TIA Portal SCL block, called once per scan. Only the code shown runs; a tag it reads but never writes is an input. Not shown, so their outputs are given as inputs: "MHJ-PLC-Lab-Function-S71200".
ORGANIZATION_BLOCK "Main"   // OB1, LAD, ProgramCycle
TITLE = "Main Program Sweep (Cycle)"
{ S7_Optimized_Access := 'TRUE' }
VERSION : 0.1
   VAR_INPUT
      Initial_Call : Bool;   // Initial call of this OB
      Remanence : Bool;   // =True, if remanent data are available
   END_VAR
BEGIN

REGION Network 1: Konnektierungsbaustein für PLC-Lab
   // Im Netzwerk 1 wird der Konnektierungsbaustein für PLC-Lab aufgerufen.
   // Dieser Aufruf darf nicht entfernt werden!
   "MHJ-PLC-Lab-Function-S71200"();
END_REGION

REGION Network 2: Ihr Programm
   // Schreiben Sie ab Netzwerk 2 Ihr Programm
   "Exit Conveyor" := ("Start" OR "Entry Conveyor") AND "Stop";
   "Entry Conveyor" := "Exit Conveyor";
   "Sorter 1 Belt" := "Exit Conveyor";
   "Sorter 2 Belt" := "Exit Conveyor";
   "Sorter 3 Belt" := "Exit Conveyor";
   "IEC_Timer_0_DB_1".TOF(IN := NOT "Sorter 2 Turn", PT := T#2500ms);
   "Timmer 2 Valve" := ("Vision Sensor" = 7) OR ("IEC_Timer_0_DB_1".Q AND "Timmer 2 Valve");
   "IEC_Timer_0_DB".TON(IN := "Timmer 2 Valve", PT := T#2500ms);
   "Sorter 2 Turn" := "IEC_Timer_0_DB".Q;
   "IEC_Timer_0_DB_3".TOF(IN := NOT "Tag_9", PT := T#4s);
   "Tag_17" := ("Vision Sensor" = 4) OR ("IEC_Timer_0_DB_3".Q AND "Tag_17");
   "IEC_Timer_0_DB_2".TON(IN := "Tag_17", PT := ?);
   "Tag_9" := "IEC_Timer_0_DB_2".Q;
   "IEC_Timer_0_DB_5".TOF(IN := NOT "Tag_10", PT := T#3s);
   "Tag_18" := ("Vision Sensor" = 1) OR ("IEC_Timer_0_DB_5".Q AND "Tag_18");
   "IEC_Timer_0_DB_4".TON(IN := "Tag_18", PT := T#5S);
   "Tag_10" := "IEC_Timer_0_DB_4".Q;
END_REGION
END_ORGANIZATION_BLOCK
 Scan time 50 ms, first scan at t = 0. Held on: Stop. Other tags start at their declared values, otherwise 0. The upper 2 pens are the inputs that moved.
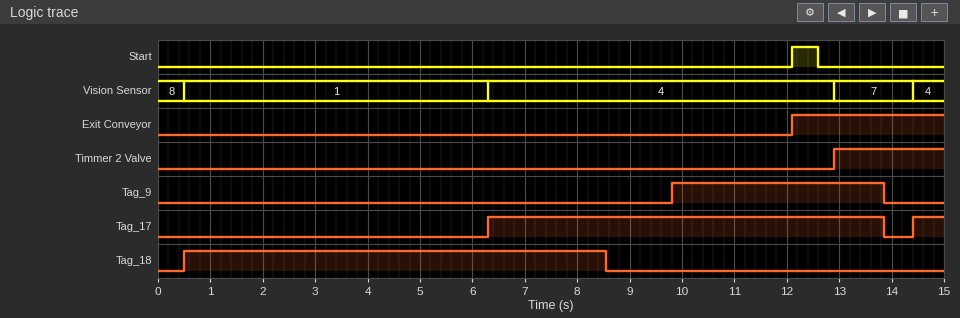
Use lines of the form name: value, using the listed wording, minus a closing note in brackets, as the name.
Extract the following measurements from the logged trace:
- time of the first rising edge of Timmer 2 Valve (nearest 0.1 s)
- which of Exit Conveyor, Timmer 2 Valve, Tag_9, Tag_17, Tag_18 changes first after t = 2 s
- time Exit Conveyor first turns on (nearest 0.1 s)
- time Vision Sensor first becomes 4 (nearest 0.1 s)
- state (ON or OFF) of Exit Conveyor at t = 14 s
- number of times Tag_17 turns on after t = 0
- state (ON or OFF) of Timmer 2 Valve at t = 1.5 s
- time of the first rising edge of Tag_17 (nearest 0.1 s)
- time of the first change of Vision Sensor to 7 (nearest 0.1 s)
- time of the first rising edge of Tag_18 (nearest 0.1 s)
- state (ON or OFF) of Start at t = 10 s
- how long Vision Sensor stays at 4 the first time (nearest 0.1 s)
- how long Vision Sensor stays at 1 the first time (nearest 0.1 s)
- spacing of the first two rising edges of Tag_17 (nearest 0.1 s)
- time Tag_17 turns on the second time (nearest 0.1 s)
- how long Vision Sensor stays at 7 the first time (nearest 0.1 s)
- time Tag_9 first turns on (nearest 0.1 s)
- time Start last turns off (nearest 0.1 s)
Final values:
time of the first rising edge of Timmer 2 Valve: 12.9 s
which of Exit Conveyor, Timmer 2 Valve, Tag_9, Tag_17, Tag_18 changes first after t = 2 s: Tag_17
time Exit Conveyor first turns on: 12.1 s
time Vision Sensor first becomes 4: 6.3 s
state (ON or OFF) of Exit Conveyor at t = 14 s: ON
number of times Tag_17 turns on after t = 0: 2
state (ON or OFF) of Timmer 2 Valve at t = 1.5 s: OFF
time of the first rising edge of Tag_17: 6.3 s
time of the first change of Vision Sensor to 7: 12.9 s
time of the first rising edge of Tag_18: 0.5 s
state (ON or OFF) of Start at t = 10 s: OFF
how long Vision Sensor stays at 4 the first time: 6.6 s
how long Vision Sensor stays at 1 the first time: 5.8 s
spacing of the first two rising edges of Tag_17: 8.1 s
time Tag_17 turns on the second time: 14.4 s
how long Vision Sensor stays at 7 the first time: 1.5 s
time Tag_9 first turns on: 9.8 s
time Start last turns off: 12.6 s
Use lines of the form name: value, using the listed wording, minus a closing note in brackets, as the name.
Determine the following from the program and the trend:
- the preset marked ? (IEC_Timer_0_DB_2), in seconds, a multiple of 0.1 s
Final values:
the preset marked ? (IEC_Timer_0_DB_2), in seconds, a multiple of 0.1 s: 3.5 s
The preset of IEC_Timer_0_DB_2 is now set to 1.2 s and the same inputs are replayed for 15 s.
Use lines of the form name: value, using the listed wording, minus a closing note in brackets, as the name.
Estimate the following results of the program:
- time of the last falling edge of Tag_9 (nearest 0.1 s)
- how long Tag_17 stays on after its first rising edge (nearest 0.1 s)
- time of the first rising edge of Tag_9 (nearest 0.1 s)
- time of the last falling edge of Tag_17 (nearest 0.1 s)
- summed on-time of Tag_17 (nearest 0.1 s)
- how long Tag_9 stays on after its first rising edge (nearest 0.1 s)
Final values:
time of the last falling edge of Tag_9: 12.9 s
how long Tag_17 stays on after its first rising edge: 6.6 s
time of the first rising edge of Tag_9: 7.5 s
time of the last falling edge of Tag_17: 12.9 s
summed on-time of Tag_17: 7.2 s
how long Tag_9 stays on after its first rising edge: 5.4 s
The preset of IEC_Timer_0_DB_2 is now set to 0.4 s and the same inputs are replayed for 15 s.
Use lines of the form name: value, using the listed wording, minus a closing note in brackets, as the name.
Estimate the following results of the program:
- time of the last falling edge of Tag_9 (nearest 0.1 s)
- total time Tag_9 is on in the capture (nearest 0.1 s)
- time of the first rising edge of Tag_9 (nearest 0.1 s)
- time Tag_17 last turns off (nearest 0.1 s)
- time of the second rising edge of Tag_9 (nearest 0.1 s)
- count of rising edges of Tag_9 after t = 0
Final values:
time of the last falling edge of Tag_9: 12.9 s
total time Tag_9 is on in the capture: 6.4 s
time of the first rising edge of Tag_9: 6.7 s
time Tag_17 last turns off: 12.9 s
time of the second rising edge of Tag_9: 14.8 s
count of rising edges of Tag_9 after t = 0: 2
